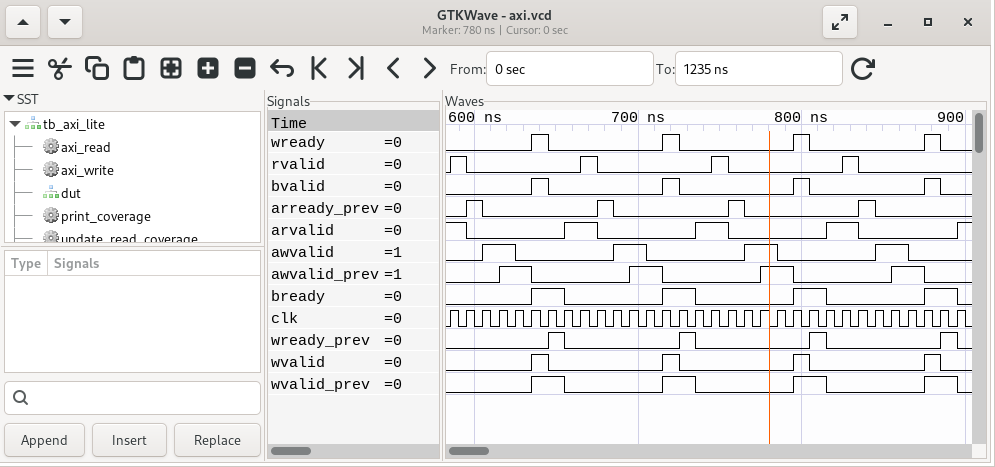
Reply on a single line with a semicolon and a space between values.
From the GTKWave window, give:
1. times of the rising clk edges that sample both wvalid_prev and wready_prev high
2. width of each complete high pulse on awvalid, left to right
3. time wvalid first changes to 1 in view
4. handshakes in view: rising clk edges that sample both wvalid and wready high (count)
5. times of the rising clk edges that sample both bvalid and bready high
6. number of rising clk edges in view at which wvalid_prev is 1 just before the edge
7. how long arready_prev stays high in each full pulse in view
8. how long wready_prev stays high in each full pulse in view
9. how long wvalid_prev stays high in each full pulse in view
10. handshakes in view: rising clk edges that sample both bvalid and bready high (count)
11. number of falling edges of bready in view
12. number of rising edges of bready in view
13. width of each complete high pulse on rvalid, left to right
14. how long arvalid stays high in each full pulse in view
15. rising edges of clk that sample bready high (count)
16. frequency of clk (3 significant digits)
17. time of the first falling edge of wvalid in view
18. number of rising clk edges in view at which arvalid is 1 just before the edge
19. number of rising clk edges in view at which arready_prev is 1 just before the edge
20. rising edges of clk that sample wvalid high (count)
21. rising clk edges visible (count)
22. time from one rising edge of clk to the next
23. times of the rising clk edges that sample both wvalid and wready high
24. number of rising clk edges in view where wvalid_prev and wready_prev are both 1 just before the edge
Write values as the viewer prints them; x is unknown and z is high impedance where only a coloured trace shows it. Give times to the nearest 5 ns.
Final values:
655 ns, 735 ns, 815 ns, 895 ns; 20 ns, 20 ns, 20 ns, 20 ns; 635 ns; 4; 645 ns, 725 ns, 805 ns, 885 ns; 8; 10 ns, 10 ns, 10 ns, 10 ns; 10 ns, 10 ns, 10 ns, 10 ns; 20 ns, 20 ns, 20 ns, 20 ns; 4; 4; 4; 10 ns, 10 ns, 10 ns, 10 ns; 20 ns, 20 ns, 20 ns; 8; 100 MHz; 645 ns; 8; 4; 4; 32; 10 ns; 645 ns, 725 ns, 805 ns, 885 ns; 4
